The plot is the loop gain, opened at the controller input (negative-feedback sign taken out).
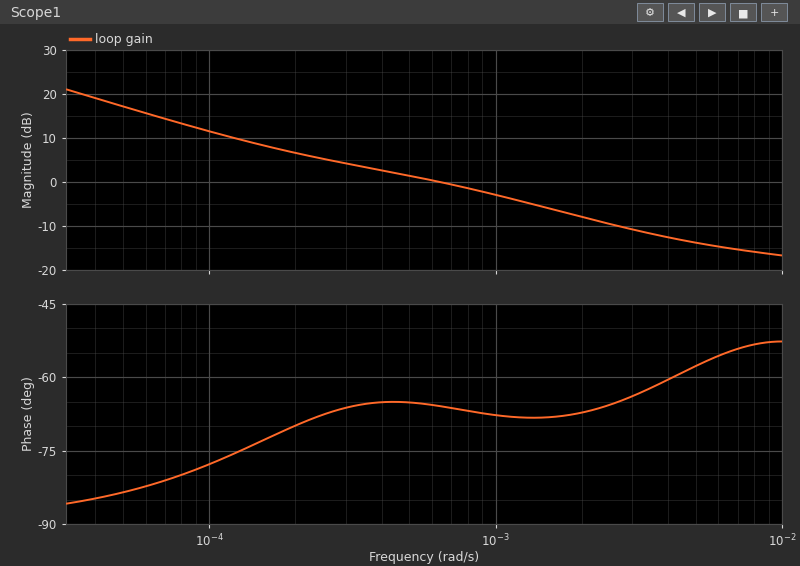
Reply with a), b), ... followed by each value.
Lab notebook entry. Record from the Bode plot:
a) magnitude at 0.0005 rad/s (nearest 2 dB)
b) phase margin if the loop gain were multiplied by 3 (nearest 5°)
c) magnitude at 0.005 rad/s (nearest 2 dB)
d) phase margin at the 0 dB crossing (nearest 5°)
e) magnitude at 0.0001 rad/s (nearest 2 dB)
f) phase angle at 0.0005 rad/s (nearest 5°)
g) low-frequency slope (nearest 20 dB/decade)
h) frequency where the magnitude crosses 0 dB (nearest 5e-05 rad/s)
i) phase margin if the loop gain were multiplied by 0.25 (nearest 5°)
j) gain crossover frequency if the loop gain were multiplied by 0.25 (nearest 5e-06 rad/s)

a) 2 dB
b) 115°
c) -14 dB
d) 115°
e) 12 dB
f) -65°
g) -20 dB/decade
h) 0.00065 rad/s
i) 100°
j) 0.000095 rad/s
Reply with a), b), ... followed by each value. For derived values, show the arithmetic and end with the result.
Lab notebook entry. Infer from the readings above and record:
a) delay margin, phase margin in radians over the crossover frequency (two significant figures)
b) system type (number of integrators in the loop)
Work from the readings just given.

a) 115 × π / 180 / 0.00065 = 3100 s
b) 1
